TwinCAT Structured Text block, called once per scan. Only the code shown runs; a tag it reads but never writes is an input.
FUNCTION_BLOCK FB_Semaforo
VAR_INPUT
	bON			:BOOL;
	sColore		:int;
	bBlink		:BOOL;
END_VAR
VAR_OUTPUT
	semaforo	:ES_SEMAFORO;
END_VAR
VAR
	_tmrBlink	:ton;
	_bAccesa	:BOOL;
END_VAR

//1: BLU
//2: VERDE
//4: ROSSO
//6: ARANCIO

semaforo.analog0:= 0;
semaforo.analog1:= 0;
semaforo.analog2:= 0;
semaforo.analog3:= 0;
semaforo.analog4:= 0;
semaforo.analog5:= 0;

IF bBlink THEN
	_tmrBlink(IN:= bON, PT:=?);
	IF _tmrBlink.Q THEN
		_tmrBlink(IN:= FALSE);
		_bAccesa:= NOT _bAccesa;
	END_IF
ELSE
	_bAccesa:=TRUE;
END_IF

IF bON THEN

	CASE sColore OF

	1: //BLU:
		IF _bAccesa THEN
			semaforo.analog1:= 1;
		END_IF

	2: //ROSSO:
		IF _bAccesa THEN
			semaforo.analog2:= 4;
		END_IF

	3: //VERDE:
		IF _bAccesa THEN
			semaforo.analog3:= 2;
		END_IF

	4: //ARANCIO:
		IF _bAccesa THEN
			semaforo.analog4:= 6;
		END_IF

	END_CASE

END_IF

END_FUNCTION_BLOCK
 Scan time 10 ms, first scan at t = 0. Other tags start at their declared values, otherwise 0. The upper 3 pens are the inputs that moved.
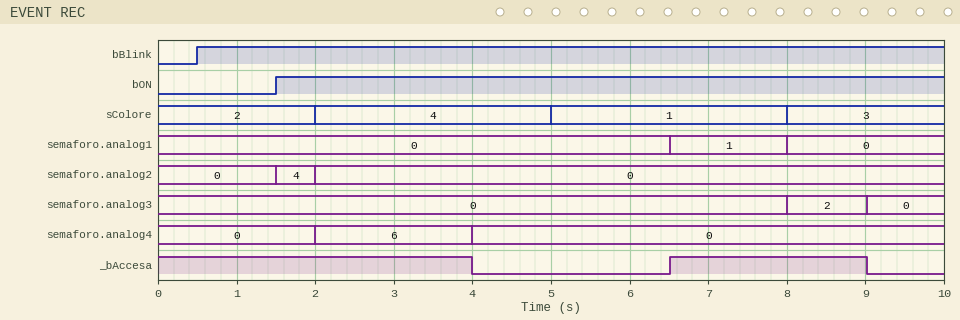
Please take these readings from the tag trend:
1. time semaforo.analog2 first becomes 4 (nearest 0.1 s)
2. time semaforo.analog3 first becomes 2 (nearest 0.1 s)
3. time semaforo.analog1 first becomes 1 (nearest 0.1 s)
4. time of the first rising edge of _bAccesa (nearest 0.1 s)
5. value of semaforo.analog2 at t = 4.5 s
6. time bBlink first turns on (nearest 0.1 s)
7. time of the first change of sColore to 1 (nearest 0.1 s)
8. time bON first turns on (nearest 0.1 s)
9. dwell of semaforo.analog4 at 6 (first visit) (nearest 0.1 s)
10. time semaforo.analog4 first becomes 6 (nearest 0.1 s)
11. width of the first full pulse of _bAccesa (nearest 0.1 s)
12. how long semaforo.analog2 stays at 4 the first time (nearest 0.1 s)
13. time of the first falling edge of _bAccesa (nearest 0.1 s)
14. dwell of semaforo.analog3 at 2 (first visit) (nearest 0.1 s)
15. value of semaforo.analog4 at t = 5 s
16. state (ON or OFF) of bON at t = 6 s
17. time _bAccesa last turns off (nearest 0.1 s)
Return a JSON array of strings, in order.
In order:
["1.5 s", "8.0 s", "6.5 s", "6.5 s", "0", "0.5 s", "5.0 s", "1.5 s", "2.0 s", "2.0 s", "2.5 s", "0.5 s", "4.0 s", "1.0 s", "0", "ON", "9.0 s"]
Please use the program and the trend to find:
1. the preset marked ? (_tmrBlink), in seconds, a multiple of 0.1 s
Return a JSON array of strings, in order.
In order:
["2.5 s"]
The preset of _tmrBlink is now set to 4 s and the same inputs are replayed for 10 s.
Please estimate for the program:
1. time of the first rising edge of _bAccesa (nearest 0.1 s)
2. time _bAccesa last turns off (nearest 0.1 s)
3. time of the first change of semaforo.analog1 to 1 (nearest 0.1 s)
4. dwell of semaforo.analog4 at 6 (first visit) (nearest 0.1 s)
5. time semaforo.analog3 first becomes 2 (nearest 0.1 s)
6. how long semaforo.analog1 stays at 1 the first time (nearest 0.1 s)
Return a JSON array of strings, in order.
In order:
["9.5 s", "5.5 s", "5.0 s", "3.0 s", "9.5 s", "0.5 s"]
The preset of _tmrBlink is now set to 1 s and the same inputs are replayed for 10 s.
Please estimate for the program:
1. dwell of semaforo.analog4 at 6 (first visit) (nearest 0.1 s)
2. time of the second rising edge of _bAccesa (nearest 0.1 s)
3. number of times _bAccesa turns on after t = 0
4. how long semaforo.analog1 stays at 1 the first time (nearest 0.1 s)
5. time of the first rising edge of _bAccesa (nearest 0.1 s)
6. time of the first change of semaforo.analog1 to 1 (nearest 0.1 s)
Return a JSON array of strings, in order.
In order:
["0.5 s", "5.5 s", "4", "1.0 s", "3.5 s", "5.5 s"]
